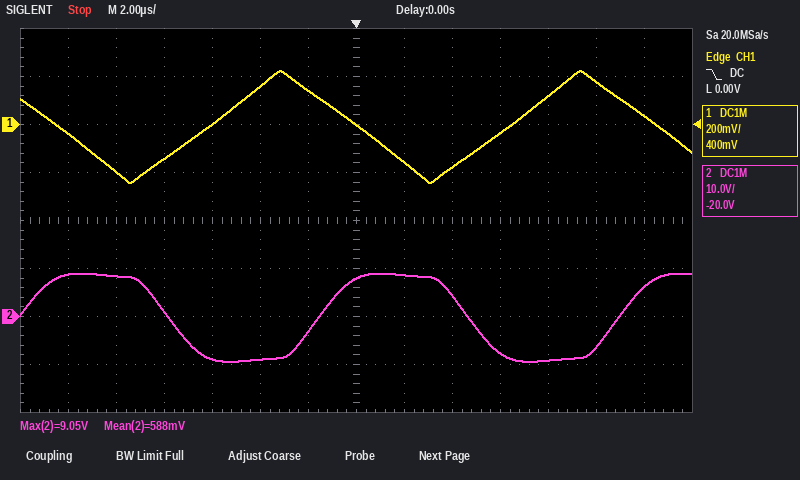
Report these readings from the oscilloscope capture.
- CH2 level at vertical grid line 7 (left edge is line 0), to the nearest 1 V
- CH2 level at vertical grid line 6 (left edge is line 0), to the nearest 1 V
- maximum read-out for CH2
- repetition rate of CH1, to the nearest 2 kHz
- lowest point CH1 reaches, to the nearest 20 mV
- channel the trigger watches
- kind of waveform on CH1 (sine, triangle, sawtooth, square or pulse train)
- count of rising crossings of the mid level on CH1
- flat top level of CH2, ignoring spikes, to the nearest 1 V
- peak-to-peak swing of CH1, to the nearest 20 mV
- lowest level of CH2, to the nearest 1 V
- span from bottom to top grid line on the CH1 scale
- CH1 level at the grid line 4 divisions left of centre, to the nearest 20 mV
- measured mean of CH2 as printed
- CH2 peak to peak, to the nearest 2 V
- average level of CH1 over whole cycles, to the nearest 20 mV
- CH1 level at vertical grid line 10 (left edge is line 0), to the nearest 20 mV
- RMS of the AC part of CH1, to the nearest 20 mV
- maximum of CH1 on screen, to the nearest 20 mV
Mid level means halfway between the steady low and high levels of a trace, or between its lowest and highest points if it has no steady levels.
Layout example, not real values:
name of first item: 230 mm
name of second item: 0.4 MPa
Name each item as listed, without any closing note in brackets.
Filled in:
CH2 level at vertical grid line 7 (left edge is line 0), to the nearest 1 V: 8 V
CH2 level at vertical grid line 6 (left edge is line 0), to the nearest 1 V: -3 V
maximum read-out for CH2: 9.05 V
repetition rate of CH1, to the nearest 2 kHz: 80 kHz
lowest point CH1 reaches, to the nearest 20 mV: -240 mV
channel the trigger watches: CH1
kind of waveform on CH1: triangle
count of rising crossings of the mid level on CH1: 2
flat top level of CH2, ignoring spikes, to the nearest 1 V: 9 V
peak-to-peak swing of CH1, to the nearest 20 mV: 460 mV
lowest level of CH2, to the nearest 1 V: -9 V
span from bottom to top grid line on the CH1 scale: 1.6 V
CH1 level at the grid line 4 divisions left of centre, to the nearest 20 mV: -140 mV
measured mean of CH2 as printed: 588 mV
CH2 peak to peak, to the nearest 2 V: 18 V
average level of CH1 over whole cycles, to the nearest 20 mV: 0 mV
CH1 level at vertical grid line 10 (left edge is line 0), to the nearest 20 mV: -40 mV
RMS of the AC part of CH1, to the nearest 20 mV: 140 mV
maximum of CH1 on screen, to the nearest 20 mV: 220 mV
